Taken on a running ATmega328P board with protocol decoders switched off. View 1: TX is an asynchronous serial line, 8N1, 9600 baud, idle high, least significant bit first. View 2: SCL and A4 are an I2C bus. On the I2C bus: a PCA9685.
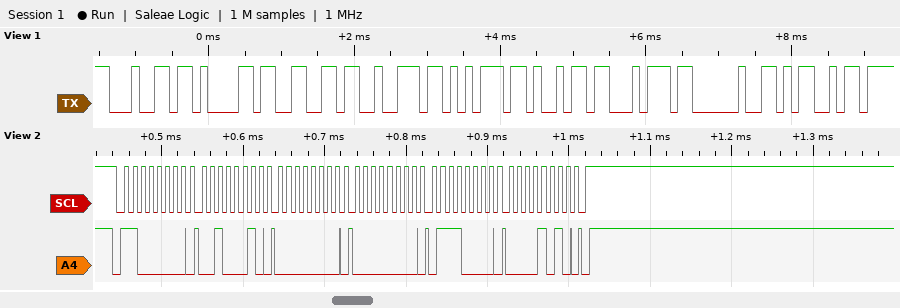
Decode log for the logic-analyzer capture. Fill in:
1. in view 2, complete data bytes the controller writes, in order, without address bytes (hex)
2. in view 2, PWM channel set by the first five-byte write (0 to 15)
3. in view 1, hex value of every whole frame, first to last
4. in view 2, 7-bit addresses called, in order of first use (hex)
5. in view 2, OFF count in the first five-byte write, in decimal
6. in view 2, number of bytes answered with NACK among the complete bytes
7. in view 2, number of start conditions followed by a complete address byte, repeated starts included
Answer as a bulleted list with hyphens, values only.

- 22 00 00 70 0A
- 7
- 0x64 0x61 0x66 0x72 0x75 0x69 0x74 0x20 0x4D
- 0x60
- 2672
- 0
- 1
